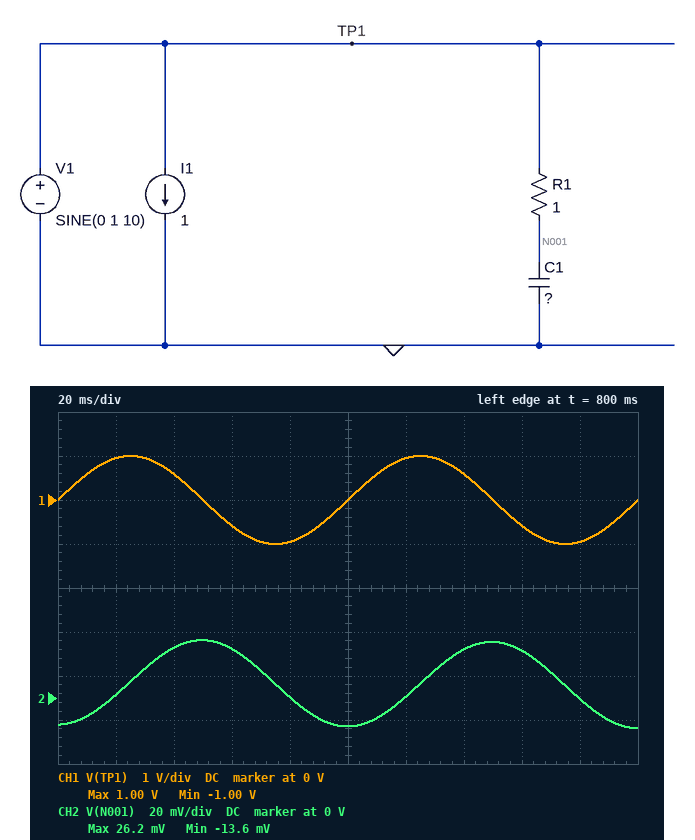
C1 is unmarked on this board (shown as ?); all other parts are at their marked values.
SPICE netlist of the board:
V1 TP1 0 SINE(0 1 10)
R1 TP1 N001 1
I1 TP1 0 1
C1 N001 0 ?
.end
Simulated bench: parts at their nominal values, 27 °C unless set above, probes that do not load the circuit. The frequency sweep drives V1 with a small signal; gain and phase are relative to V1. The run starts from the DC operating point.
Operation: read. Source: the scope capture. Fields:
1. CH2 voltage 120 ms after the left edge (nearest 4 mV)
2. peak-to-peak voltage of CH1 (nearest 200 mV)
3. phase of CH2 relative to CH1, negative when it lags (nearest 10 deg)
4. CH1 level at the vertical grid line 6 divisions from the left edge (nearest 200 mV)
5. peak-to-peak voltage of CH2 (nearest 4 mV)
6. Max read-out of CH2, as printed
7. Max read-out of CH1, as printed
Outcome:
0 V
2.0 V
-90 deg
1.0 V
40 mV
26.2 mV
1.00 V
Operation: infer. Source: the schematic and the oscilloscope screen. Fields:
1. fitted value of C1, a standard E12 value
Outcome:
820 mF
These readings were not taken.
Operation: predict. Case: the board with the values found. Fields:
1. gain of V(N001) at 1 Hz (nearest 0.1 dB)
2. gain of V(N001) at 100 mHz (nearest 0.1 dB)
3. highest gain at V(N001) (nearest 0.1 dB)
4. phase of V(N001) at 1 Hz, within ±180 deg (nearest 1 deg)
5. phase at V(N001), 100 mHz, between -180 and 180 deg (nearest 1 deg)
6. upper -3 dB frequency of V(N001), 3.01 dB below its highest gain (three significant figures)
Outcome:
-14.4 dB
-1.0 dB
0 dB
-79 deg
-27 deg
194 mHz
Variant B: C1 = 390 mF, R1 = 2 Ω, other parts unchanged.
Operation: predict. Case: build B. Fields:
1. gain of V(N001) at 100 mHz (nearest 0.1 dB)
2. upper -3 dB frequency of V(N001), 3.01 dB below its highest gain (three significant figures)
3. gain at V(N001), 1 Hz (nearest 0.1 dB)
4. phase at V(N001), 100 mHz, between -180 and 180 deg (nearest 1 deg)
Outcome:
-0.9 dB
204 mHz
-14.0 dB
-26 deg
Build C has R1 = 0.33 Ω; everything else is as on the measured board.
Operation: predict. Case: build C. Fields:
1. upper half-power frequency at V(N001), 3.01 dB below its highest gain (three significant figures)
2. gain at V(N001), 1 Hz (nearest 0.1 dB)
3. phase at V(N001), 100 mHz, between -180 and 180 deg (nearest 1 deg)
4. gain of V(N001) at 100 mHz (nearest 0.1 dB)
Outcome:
588 mHz
-5.9 dB
-10 deg
-0.1 dB
